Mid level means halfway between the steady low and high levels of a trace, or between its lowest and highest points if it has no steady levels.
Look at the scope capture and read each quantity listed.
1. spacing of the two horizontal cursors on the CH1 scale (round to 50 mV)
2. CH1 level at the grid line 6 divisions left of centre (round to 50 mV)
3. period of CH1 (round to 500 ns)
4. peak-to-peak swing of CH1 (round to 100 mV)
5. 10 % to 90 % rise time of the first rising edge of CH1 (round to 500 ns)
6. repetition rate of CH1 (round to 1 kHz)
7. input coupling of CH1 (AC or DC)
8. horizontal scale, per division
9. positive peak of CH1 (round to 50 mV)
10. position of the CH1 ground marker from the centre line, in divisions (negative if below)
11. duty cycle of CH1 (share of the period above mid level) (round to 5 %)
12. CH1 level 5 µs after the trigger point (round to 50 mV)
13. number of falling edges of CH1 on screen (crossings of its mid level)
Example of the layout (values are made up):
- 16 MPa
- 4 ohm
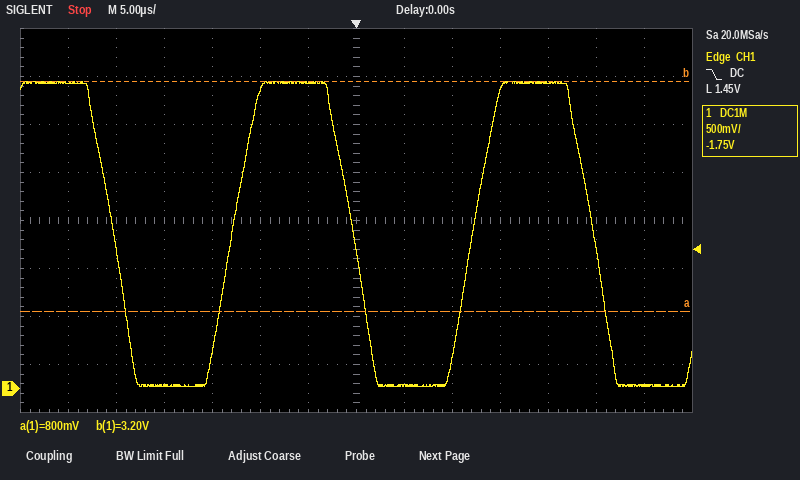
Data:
- 2.40 V
- 3.20 V
- 25.0 µs
- 3.20 V
- 4.5 µs
- 40 kHz
- DC
- 5 µs
- 3.20 V
- -3.5 div
- 50 %
- 50 mV
- 3
